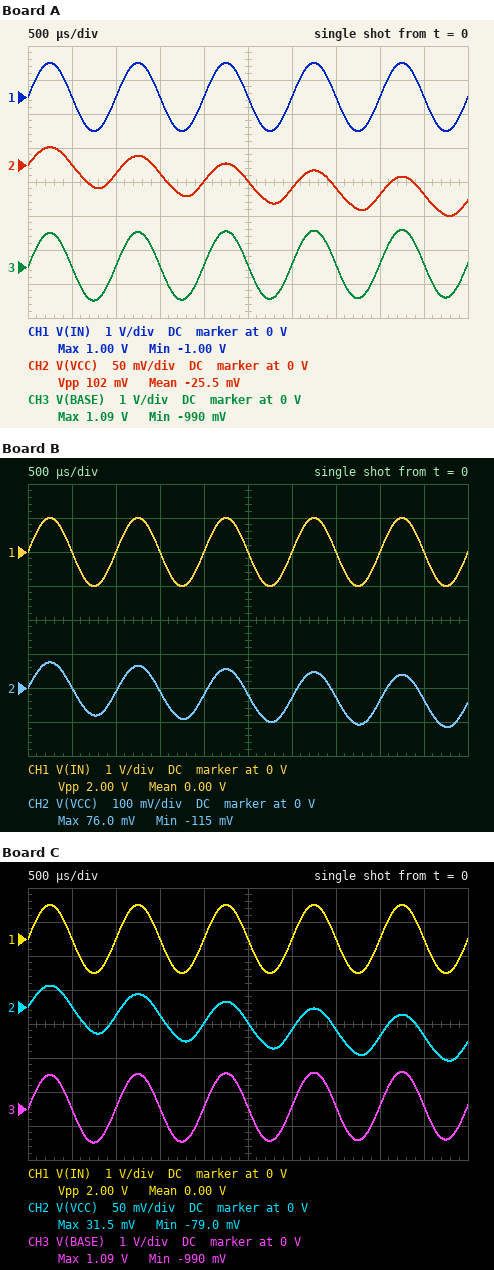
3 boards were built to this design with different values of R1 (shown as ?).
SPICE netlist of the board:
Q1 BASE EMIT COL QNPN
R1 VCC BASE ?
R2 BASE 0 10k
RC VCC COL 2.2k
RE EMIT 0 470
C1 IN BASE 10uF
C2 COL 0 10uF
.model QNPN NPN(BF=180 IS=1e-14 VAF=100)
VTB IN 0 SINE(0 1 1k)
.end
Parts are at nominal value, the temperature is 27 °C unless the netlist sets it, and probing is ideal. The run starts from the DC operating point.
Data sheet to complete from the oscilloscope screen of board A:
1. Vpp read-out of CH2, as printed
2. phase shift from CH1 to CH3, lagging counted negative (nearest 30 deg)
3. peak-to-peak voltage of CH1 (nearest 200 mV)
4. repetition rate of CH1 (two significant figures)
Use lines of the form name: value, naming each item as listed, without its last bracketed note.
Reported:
Vpp read-out of CH2, as printed: 102 mV
phase shift from CH1 to CH3, lagging counted negative: 0 deg
peak-to-peak voltage of CH1: 2.0 V
repetition rate of CH1: 1.0 kHz
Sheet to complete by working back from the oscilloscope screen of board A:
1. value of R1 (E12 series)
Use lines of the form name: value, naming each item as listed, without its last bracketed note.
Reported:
value of R1: 82 kΩ
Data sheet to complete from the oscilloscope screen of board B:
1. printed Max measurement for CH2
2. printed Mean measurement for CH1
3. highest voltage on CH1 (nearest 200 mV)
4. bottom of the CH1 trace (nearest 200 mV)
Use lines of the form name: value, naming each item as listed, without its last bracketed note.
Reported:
printed Max measurement for CH2: 76.0 mV
printed Mean measurement for CH1: 0.00 V
highest voltage on CH1: 1.0 V
bottom of the CH1 trace: -1.0 V
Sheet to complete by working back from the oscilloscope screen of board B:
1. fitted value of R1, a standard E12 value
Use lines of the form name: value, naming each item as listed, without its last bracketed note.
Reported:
fitted value of R1, a standard E12 value: 27 kΩ
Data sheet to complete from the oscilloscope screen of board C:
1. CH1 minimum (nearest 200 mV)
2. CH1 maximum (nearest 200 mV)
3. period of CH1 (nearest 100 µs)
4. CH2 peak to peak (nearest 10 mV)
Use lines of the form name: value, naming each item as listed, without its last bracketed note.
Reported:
CH1 minimum: -1.0 V
CH1 maximum: 1.0 V
period of CH1: 1.0 ms
CH2 peak to peak: 110 mV
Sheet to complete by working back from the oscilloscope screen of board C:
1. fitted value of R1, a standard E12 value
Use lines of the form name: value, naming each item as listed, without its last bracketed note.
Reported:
fitted value of R1, a standard E12 value: 68 kΩ
